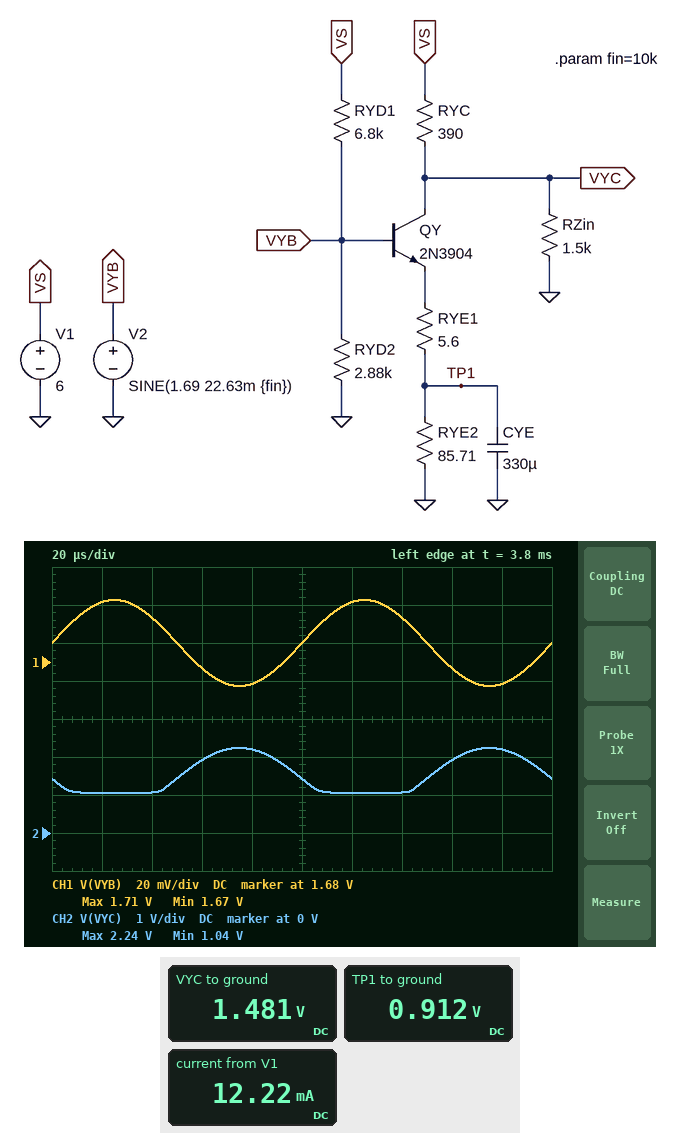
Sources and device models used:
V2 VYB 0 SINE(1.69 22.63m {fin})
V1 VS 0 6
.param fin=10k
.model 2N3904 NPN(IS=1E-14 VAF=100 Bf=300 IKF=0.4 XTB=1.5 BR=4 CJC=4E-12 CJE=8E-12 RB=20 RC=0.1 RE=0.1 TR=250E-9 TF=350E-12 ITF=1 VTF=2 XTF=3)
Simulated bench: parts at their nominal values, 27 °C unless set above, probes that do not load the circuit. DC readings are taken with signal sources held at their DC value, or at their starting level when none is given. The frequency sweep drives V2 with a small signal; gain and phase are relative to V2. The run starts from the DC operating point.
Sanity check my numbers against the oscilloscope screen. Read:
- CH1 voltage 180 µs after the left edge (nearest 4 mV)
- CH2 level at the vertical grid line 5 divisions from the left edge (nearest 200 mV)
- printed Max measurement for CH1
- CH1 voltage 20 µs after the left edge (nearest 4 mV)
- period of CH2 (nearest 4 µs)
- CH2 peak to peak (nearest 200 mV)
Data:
1.668 V
1.4 V
1.71 V
1.712 V
100 µs
1.2 V
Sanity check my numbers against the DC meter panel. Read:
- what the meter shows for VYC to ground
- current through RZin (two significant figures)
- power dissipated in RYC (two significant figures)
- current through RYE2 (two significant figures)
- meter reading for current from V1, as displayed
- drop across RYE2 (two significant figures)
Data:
1.481 V
990 µA
52 mW
11 mA
12.22 mA
910 mV
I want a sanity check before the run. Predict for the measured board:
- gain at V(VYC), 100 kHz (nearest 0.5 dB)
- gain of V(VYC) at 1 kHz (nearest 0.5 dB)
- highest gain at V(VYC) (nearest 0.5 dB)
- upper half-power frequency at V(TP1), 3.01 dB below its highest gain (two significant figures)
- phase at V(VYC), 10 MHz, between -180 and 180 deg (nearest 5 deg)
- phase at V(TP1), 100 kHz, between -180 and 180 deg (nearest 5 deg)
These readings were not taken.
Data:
31.5 dB
31.5 dB
31.5 dB
63 Hz
160 deg
-90 deg
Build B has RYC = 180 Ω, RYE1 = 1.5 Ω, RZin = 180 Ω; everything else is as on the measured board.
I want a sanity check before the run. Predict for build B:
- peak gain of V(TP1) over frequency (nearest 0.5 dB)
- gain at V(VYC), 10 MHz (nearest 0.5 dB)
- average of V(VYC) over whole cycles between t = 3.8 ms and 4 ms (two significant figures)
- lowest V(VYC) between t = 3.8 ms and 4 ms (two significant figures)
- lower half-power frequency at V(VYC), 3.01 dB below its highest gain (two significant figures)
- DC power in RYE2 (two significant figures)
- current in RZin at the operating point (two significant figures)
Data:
-0.5 dB
26.5 dB
2.0 V
1.5 V
120 Hz
11 mW
11 mA
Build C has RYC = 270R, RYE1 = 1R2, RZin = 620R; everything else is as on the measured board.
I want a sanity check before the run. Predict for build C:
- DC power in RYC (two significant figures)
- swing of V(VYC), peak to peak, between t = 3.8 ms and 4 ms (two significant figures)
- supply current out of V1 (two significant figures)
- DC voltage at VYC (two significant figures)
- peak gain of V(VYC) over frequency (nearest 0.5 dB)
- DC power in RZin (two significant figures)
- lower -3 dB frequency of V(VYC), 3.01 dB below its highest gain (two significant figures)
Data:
57 mW
2.0 V
15 mA
2.1 V
34.0 dB
7.0 mW
130 Hz
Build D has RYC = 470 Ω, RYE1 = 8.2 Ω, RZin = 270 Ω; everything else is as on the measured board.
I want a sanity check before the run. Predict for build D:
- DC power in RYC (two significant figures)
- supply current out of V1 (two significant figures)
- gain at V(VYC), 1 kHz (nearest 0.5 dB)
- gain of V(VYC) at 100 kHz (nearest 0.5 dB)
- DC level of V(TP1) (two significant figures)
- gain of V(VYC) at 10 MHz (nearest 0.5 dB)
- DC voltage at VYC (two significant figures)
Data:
55 mW
11 mA
-19.0 dB
-15.0 dB
830 mV
-10.0 dB
930 mV
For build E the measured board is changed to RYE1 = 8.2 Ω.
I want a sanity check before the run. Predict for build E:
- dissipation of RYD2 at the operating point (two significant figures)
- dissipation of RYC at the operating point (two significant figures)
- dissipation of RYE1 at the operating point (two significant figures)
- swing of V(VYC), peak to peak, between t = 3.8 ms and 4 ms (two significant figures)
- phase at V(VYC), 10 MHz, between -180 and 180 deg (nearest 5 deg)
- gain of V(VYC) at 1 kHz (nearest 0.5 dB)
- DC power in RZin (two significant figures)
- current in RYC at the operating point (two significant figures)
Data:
990 µW
50 mW
880 µW
1.1 V
165 deg
29.0 dB
1.6 mW
11 mA
